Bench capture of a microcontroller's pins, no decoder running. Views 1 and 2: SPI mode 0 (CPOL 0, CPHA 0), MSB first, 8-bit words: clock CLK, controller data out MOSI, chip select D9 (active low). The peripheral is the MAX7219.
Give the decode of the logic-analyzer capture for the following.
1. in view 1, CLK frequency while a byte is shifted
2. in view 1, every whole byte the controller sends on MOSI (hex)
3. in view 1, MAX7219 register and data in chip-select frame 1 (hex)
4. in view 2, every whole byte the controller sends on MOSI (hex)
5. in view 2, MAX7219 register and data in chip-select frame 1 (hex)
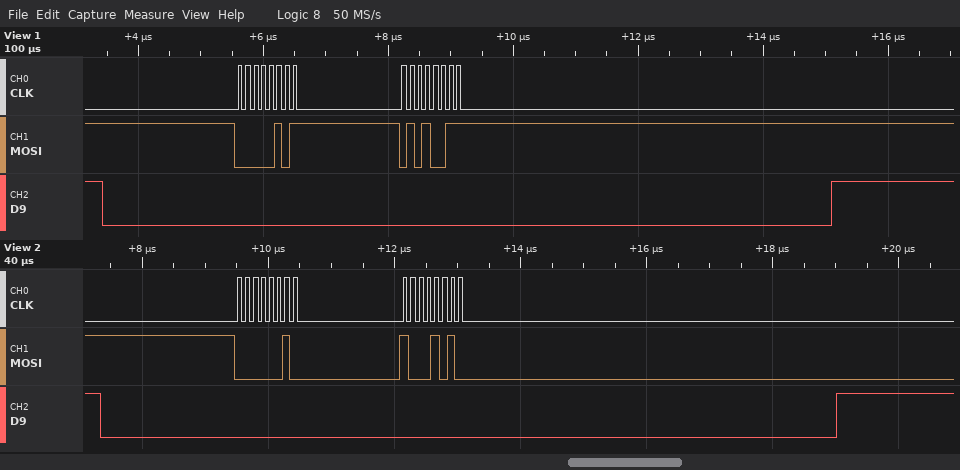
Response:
8 MHz
05 53
register 0x5, data 0x53
02 8A
register 0x2, data 0x8A
